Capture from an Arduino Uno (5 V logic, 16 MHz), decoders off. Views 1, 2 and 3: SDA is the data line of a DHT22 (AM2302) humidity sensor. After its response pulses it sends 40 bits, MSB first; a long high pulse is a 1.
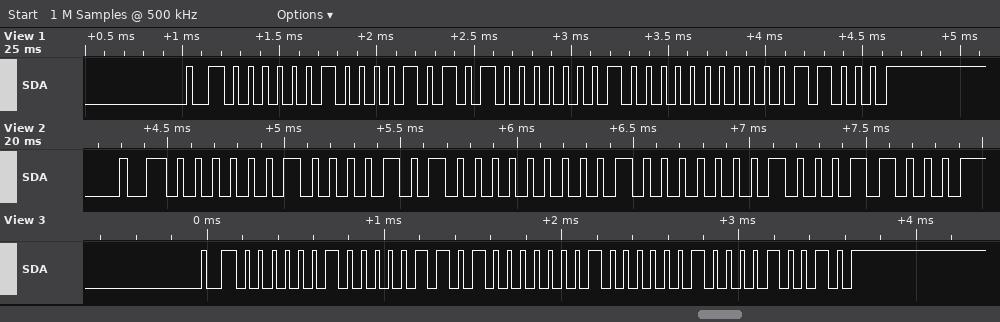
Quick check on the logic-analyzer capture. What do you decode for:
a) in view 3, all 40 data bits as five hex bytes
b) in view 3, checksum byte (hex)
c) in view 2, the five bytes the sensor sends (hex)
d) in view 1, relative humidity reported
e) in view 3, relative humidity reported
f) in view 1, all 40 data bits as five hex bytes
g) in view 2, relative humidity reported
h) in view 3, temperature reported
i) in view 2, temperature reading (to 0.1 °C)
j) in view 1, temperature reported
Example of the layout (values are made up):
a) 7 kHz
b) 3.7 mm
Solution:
a) 02 0D 01 02 12
b) 0x12
c) 02 14 01 01 18
d) 53.3 %
e) 52.5 %
f) 02 15 01 00 18
g) 53.2 %
h) 25.8 °C
i) 25.7 °C
j) 25.6 °C
